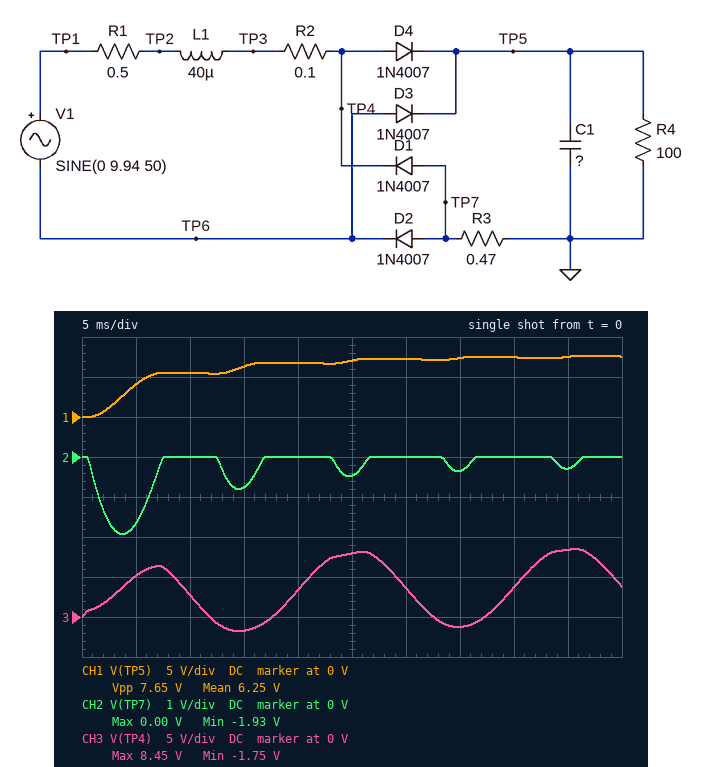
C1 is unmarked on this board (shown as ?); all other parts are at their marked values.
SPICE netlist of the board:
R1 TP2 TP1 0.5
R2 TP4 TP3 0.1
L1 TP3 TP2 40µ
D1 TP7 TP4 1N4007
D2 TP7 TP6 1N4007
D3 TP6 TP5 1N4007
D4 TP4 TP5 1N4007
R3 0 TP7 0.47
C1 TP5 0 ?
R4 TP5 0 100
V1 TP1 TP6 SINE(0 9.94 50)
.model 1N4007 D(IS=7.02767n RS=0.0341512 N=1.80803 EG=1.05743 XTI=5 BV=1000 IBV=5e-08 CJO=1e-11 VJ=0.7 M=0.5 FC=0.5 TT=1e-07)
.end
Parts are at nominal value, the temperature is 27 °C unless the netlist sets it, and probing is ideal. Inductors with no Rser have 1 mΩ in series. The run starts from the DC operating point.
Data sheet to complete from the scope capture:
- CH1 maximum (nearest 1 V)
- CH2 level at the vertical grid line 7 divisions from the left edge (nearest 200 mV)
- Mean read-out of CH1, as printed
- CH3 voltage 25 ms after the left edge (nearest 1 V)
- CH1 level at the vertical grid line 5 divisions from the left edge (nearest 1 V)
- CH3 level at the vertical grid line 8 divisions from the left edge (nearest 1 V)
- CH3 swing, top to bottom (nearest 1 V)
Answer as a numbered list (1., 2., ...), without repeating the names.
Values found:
1. 8 V
2. -400 mV
3. 6.25 V
4. 8 V
5. 7 V
6. 4 V
7. 10 V
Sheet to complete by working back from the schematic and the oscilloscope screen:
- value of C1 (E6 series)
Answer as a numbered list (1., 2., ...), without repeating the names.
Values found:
1. 3.3 mF
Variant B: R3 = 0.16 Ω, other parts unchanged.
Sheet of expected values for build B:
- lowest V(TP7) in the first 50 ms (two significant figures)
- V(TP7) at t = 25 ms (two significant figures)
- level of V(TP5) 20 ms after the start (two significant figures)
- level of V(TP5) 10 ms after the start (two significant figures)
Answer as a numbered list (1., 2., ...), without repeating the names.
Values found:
1. -780 mV
2. -150 mV
3. 7.2 V
4. 6.2 V
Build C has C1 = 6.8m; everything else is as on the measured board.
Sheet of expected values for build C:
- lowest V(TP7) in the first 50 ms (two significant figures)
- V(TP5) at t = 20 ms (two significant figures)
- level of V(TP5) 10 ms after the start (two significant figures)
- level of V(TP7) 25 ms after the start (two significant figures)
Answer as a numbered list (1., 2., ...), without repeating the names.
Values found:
1. -2.4 V
2. 5.3 V
3. 3.7 V
4. -950 mV
